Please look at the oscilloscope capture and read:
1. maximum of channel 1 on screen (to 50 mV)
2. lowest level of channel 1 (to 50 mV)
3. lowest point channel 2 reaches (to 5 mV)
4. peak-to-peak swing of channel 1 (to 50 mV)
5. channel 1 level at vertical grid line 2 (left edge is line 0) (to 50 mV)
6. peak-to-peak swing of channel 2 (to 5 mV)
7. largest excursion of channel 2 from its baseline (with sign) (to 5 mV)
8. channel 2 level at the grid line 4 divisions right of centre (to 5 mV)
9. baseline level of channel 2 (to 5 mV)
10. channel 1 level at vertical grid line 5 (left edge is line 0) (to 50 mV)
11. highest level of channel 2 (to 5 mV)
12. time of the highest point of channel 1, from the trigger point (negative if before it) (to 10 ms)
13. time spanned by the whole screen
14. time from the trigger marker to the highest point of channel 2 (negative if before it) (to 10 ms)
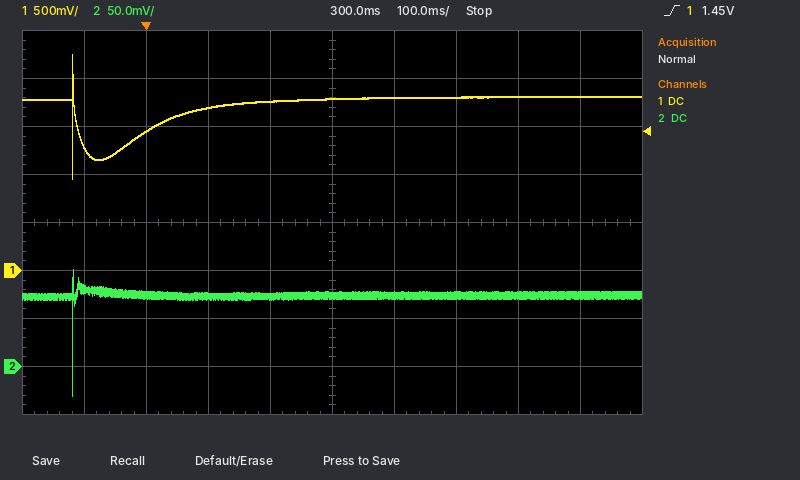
2.25 V
950 mV
-30 mV
1.30 V
1.45 V
130 mV
-105 mV
75 mV
75 mV
1.80 V
100 mV
-120 ms
1 s
-120 ms
